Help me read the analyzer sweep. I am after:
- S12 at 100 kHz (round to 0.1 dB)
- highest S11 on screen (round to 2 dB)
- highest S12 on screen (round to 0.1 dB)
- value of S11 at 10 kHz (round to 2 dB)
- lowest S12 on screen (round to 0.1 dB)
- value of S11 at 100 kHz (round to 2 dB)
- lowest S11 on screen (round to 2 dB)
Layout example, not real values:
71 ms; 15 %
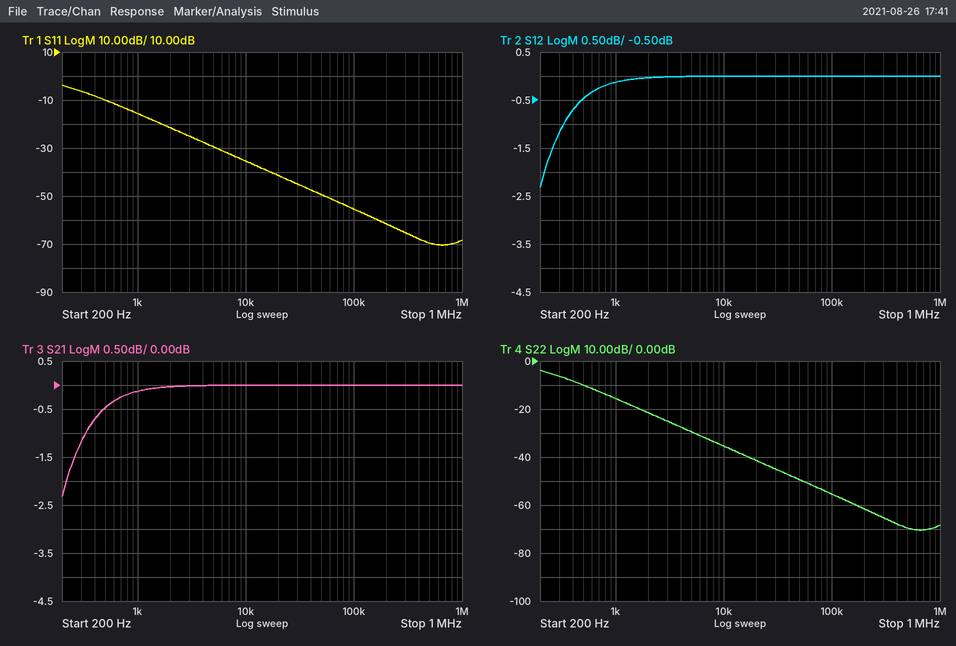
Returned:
0.0 dB; -4 dB; 0.0 dB; -36 dB; -2.3 dB; -56 dB; -70 dB
